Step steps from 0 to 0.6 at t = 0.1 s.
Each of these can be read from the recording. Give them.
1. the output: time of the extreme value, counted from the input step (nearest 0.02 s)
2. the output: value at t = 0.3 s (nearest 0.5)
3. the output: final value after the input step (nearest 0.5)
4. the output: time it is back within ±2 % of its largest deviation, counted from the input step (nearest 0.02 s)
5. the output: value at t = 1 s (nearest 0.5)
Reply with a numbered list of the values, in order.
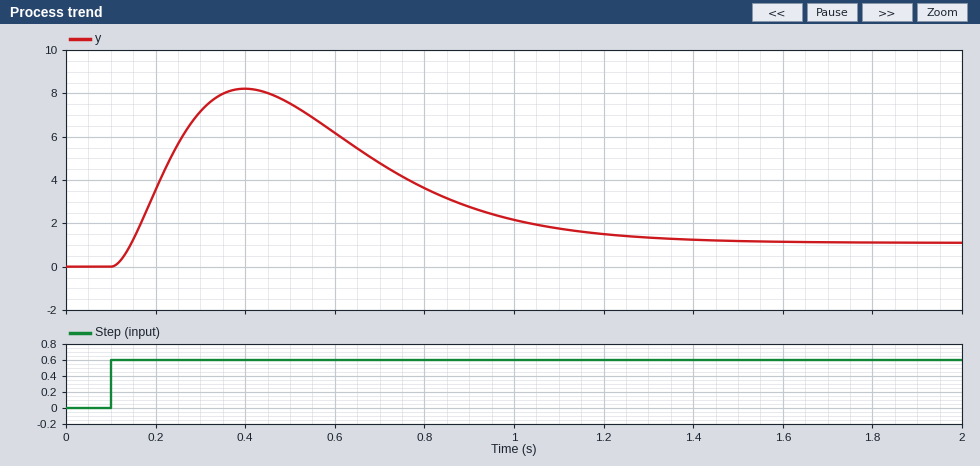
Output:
1. 0.30 s
2. 7.0
3. 1.0
4. 1.28 s
5. 2.0
